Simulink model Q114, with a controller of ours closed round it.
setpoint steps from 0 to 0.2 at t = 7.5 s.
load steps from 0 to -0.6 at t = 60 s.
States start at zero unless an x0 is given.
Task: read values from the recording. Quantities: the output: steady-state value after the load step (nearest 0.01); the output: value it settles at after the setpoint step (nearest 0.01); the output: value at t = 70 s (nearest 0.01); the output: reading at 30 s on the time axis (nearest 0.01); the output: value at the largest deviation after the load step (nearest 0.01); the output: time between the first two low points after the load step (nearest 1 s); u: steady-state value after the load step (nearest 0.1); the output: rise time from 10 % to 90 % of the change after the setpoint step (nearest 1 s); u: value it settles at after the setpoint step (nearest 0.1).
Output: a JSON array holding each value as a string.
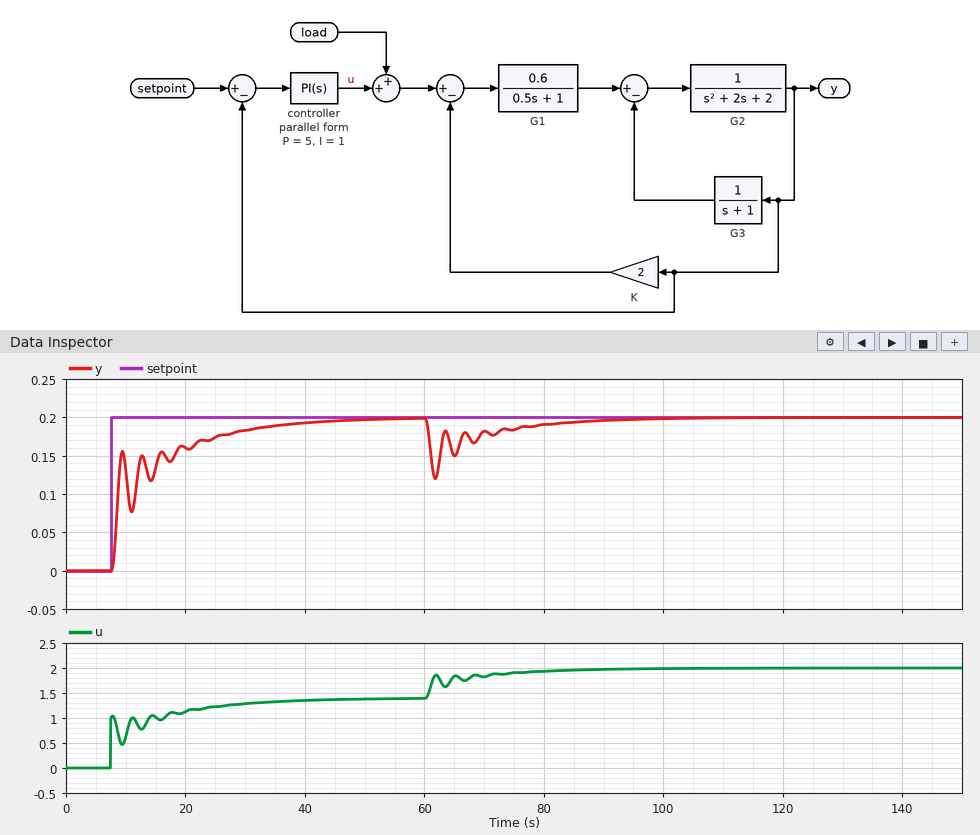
["0.20", "0.20", "0.18", "0.18", "0.12", "3 s", "2.0", "20 s", "1.4"]
